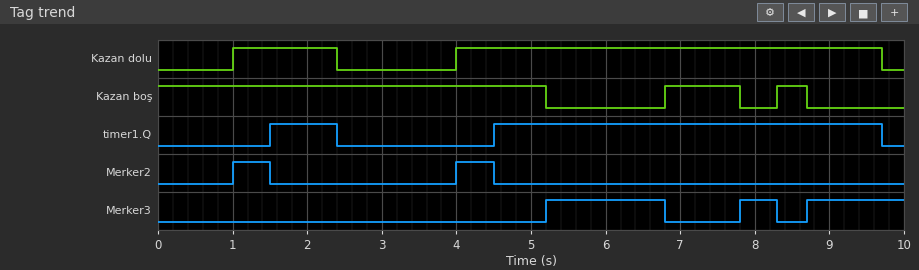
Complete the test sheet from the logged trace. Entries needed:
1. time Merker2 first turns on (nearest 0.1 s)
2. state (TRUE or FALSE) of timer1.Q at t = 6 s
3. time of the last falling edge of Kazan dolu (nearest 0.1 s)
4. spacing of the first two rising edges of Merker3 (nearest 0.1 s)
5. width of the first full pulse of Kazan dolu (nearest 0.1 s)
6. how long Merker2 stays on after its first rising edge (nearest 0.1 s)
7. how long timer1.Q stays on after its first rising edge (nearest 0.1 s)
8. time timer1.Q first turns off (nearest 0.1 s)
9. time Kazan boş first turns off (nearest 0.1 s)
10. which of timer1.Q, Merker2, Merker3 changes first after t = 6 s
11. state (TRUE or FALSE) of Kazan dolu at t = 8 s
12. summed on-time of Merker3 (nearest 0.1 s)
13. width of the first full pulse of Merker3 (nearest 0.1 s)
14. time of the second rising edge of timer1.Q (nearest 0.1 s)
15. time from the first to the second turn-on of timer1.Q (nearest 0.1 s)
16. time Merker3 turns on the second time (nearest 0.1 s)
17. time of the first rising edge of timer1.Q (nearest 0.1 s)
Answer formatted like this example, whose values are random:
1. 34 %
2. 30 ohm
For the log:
1. 1.0 s
2. TRUE
3. 9.7 s
4. 2.6 s
5. 1.4 s
6. 0.5 s
7. 0.9 s
8. 2.4 s
9. 5.2 s
10. Merker3
11. TRUE
12. 3.4 s
13. 1.6 s
14. 4.5 s
15. 3.0 s
16. 7.8 s
17. 1.5 s
